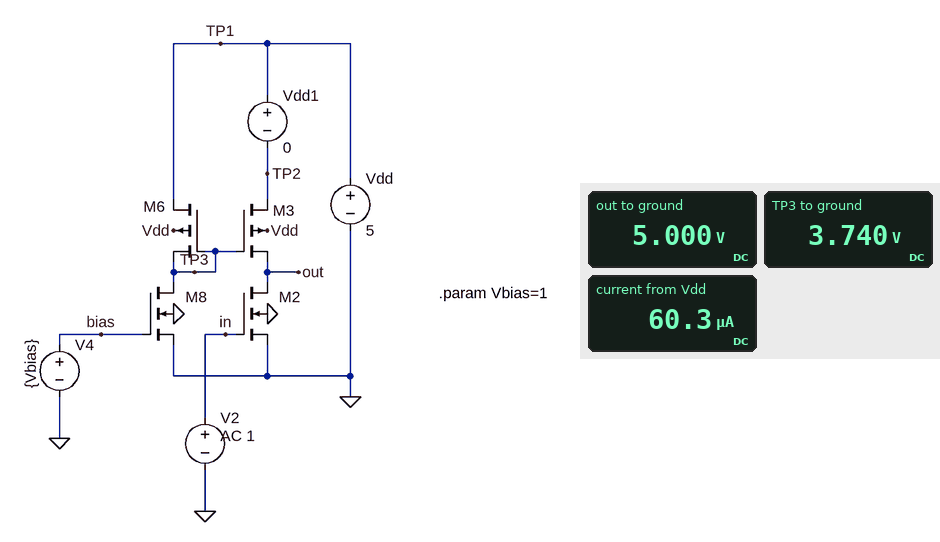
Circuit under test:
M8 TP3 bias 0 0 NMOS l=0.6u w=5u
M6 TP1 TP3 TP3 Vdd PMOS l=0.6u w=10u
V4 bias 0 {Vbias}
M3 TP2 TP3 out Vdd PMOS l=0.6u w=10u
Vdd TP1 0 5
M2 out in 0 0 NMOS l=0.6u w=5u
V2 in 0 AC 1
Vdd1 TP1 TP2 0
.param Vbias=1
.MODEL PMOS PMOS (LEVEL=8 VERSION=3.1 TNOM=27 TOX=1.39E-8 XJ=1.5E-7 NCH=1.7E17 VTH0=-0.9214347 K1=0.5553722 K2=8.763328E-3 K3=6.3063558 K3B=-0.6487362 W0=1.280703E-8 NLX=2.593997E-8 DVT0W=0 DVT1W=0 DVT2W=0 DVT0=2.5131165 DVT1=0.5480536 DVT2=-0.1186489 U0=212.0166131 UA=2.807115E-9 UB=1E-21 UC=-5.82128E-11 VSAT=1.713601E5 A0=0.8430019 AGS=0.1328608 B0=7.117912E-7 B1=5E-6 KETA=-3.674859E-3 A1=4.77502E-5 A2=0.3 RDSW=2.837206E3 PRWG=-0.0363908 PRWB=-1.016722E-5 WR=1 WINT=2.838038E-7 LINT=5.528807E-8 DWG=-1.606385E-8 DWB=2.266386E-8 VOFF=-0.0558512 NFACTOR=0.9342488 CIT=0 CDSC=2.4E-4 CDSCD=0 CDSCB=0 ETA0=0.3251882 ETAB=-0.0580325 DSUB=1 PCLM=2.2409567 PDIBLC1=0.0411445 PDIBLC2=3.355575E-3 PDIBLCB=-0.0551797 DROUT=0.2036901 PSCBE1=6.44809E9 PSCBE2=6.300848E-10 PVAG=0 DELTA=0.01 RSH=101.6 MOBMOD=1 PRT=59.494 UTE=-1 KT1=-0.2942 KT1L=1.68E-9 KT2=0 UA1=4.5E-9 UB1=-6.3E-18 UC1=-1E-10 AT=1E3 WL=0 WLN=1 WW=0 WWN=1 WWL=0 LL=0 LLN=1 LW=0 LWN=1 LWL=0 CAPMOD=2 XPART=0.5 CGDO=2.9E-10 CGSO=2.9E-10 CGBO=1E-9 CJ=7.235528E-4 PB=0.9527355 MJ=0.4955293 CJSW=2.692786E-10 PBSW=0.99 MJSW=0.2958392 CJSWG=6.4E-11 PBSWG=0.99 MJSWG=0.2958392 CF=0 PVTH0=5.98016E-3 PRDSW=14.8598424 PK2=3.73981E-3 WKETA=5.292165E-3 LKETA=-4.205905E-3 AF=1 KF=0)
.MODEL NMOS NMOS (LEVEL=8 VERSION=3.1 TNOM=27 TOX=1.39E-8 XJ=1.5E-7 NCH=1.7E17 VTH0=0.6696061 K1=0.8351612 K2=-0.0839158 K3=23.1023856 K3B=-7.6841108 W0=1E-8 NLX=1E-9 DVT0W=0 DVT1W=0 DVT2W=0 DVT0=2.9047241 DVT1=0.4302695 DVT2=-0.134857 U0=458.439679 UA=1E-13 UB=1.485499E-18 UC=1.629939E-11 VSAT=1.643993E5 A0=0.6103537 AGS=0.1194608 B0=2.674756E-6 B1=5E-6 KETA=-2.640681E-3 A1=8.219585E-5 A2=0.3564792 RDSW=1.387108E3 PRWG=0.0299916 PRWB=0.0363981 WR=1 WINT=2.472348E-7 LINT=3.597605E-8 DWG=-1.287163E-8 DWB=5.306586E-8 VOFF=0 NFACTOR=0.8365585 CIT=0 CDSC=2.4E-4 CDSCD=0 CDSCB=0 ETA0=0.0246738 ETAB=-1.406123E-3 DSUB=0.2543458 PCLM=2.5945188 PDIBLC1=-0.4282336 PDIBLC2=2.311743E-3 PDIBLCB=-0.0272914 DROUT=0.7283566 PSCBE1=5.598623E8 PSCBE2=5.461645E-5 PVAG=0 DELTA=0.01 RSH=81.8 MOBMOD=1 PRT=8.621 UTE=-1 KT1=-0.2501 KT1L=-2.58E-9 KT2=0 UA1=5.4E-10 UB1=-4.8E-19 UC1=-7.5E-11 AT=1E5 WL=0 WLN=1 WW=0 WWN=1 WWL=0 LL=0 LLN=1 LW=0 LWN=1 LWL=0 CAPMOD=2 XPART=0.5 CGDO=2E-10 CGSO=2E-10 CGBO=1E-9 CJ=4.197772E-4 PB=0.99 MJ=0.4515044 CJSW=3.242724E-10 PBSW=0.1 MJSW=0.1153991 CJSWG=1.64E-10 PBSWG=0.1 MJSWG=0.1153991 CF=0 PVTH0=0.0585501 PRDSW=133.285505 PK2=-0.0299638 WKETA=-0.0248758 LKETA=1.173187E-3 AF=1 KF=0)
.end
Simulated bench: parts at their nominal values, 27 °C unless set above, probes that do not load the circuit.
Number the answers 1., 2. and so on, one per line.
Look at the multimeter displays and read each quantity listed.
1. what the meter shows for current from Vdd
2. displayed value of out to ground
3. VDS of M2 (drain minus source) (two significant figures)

1. 60.3 µA
2. 5.000 V
3. 5.0 V
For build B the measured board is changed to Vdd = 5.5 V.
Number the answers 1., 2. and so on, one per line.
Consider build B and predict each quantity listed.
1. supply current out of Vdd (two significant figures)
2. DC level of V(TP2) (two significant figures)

1. 63 µA
2. 5.5 V
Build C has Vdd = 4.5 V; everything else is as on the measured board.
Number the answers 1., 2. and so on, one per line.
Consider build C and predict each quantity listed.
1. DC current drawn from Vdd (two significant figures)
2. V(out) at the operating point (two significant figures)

1. 58 µA
2. 4.5 V
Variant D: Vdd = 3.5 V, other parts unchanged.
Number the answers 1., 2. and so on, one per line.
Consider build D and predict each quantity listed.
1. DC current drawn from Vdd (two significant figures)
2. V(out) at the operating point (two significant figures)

1. 54 µA
2. 3.5 V
